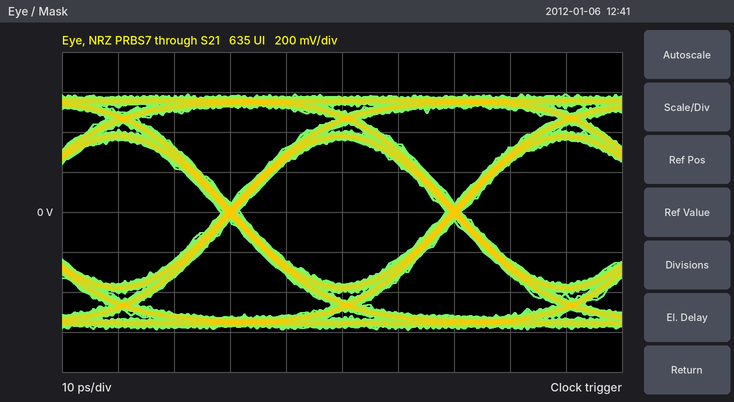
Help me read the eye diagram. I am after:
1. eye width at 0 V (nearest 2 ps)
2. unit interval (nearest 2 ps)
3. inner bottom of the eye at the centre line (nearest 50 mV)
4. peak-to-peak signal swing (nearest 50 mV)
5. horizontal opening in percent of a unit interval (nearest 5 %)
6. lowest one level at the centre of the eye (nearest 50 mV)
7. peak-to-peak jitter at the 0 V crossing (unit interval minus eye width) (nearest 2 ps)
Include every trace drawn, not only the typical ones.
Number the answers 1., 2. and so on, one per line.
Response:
1. 36 ps
2. 40 ps
3. -350 mV
4. 1.20 V
5. 90 %
6. 350 mV
7. 4 ps
